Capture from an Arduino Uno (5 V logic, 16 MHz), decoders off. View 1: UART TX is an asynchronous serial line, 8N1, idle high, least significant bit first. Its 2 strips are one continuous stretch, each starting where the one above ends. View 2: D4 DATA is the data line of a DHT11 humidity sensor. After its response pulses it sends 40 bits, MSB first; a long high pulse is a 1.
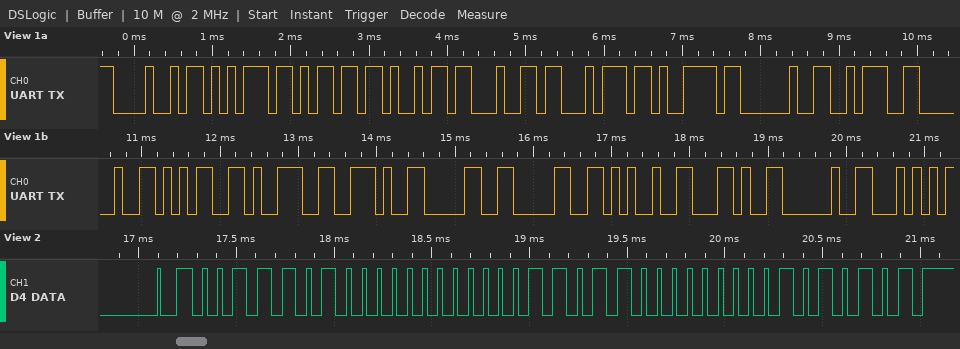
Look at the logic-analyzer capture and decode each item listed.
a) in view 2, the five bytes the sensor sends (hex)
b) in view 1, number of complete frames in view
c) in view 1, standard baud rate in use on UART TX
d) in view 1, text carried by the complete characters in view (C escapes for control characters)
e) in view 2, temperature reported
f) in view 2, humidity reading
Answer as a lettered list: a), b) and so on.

a) 3A 00 1B 00 55
b) 19
c) 9600 baud
d) "Humidty : 59.00%, T"
e) 27.0 °C
f) 58 %
